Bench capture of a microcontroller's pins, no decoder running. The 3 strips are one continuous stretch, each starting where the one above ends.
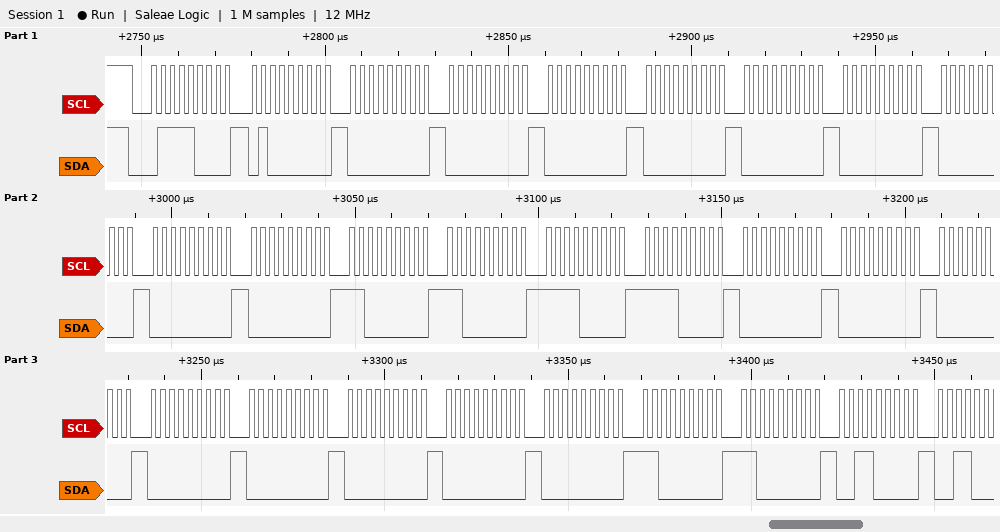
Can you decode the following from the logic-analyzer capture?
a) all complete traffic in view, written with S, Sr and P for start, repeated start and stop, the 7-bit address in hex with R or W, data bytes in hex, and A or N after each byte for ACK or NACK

S 3CW A 40 A 00 A 00 A 00 A 00 A 00 A 00 A 00 A 00 A 00 A C0 A C0 A F0 A F0 A 00 A 00 A 00 A 00 A 00 A 00 A 00 A 00 A C0 A C0 A 30 A
